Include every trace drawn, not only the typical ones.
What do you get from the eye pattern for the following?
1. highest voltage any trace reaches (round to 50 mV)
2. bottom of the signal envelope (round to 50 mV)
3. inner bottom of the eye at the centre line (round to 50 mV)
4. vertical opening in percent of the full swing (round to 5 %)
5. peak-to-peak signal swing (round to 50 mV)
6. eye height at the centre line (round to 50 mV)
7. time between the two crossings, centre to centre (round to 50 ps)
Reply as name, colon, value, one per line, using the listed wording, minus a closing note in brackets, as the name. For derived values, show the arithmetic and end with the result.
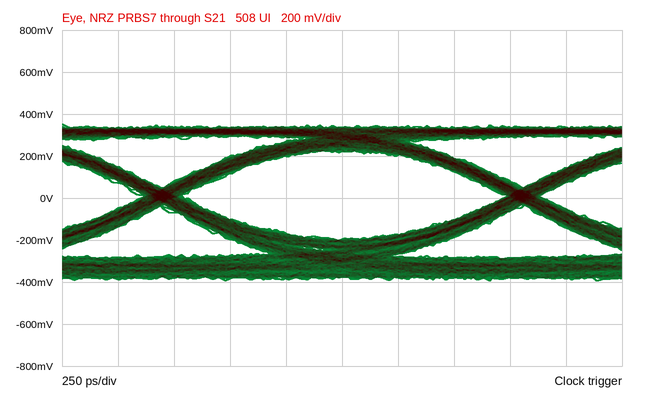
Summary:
highest voltage any trace reaches: 350 mV
bottom of the signal envelope: -400 mV
inner bottom of the eye at the centre line: -200 mV
vertical opening in percent of the full swing: 400 mV / 750 mV ≈ 53.3 %, so 55 % to the nearest 5 %
peak-to-peak signal swing: 750 mV
eye height at the centre line: 400 mV
time between the two crossings, centre to centre: 1.60 ns
